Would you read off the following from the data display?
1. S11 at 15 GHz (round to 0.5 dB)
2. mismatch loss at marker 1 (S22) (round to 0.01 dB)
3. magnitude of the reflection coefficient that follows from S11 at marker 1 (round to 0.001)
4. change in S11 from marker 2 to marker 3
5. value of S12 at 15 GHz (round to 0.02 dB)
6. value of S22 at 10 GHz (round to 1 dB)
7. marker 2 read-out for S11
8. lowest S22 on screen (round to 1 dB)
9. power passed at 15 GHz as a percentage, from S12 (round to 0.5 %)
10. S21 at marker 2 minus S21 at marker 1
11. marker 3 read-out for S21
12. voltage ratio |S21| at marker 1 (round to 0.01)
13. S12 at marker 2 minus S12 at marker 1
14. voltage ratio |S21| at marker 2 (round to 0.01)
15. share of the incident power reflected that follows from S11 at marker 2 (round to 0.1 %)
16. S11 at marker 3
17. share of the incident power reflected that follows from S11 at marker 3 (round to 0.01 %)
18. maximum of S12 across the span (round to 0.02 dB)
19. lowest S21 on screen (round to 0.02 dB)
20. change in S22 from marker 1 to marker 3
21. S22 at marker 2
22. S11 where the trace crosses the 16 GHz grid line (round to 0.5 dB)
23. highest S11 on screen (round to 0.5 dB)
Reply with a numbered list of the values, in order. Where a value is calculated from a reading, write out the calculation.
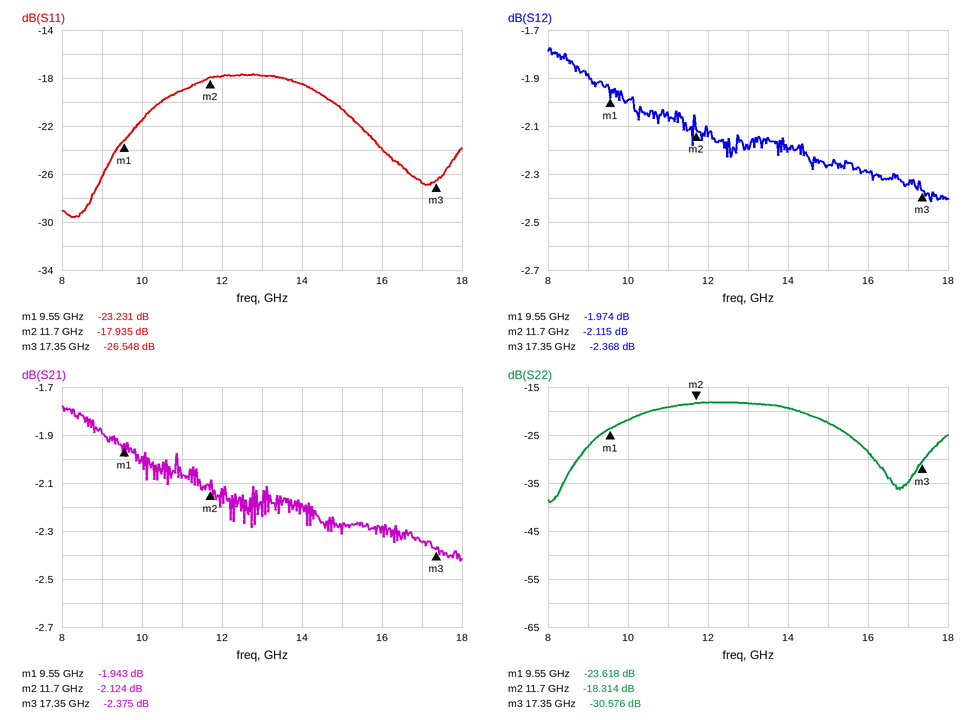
1. -20.5 dB
2. −10 log10(1 − 10^(-23.618/10)) ≈ 0.02 dB
3. 10^(-23.231/20) ≈ 0.069
4. -26.548 − (-17.935) = -8.613 dB
5. -2.26 dB
6. -22 dB
7. -17.935 dB
8. -39 dB
9. 10^(-2.26/10) ≈ 59.4 %, so 59.5 % to the nearest 0.5 %
10. -2.124 − (-1.943) = -0.181 dB
11. -2.375 dB
12. 10^(-1.943/20) ≈ 0.80
13. -2.115 − (-1.974) = -0.141 dB
14. 10^(-2.124/20) ≈ 0.78
15. 10^(-17.935/10) ≈ 1.6 %
16. -26.548 dB
17. 10^(-26.548/10) ≈ 0.22 %
18. -1.78 dB
19. -2.42 dB
20. -30.576 − (-23.618) = -6.958 dB
21. -18.314 dB
22. -24.0 dB
23. -17.5 dB
